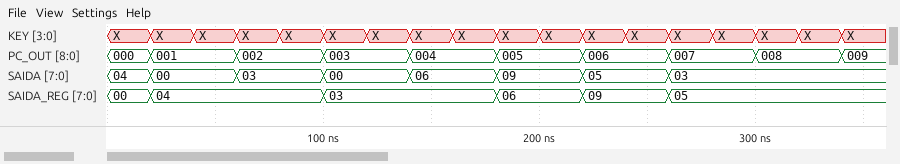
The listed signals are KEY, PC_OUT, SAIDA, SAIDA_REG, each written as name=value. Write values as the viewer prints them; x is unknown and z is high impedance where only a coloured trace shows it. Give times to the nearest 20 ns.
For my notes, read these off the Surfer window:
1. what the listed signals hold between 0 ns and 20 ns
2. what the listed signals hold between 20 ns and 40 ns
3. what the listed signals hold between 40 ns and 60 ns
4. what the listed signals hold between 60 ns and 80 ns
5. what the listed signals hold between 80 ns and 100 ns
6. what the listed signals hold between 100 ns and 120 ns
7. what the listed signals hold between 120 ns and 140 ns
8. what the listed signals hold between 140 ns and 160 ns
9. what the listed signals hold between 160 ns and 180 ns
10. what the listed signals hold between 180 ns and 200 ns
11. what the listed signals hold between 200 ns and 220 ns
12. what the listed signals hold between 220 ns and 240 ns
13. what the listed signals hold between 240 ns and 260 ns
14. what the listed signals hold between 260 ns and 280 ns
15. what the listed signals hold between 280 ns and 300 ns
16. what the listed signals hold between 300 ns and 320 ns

KEY=X, PC_OUT=000, SAIDA=04, SAIDA_REG=00
KEY=X, PC_OUT=001, SAIDA=00, SAIDA_REG=04
KEY=X, PC_OUT=001, SAIDA=00, SAIDA_REG=04
KEY=X, PC_OUT=002, SAIDA=03, SAIDA_REG=04
KEY=X, PC_OUT=002, SAIDA=03, SAIDA_REG=04
KEY=X, PC_OUT=003, SAIDA=00, SAIDA_REG=03
KEY=X, PC_OUT=003, SAIDA=00, SAIDA_REG=03
KEY=X, PC_OUT=004, SAIDA=06, SAIDA_REG=03
KEY=X, PC_OUT=004, SAIDA=06, SAIDA_REG=03
KEY=X, PC_OUT=005, SAIDA=09, SAIDA_REG=06
KEY=X, PC_OUT=005, SAIDA=09, SAIDA_REG=06
KEY=X, PC_OUT=006, SAIDA=05, SAIDA_REG=09
KEY=X, PC_OUT=006, SAIDA=05, SAIDA_REG=09
KEY=X, PC_OUT=007, SAIDA=03, SAIDA_REG=05
KEY=X, PC_OUT=007, SAIDA=03, SAIDA_REG=05
KEY=X, PC_OUT=008, SAIDA=03, SAIDA_REG=05
